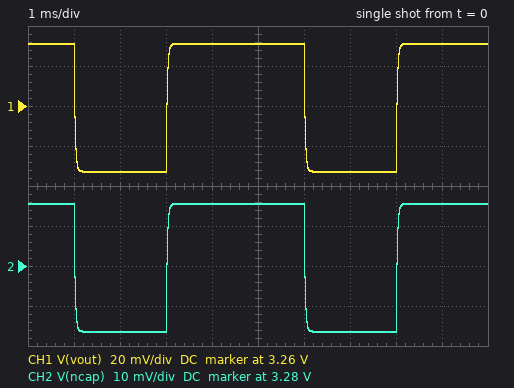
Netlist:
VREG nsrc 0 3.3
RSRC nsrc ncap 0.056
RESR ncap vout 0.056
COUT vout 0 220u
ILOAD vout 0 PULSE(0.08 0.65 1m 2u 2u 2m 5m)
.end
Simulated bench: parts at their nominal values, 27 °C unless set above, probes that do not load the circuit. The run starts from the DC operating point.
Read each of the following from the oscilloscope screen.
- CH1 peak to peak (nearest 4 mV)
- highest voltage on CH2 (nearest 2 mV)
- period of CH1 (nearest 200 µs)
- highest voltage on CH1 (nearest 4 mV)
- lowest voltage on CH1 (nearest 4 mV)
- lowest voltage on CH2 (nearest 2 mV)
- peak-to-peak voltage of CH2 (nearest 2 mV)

64 mV
3.296 V
5.0 ms
3.292 V
3.228 V
3.264 V
32 mV
